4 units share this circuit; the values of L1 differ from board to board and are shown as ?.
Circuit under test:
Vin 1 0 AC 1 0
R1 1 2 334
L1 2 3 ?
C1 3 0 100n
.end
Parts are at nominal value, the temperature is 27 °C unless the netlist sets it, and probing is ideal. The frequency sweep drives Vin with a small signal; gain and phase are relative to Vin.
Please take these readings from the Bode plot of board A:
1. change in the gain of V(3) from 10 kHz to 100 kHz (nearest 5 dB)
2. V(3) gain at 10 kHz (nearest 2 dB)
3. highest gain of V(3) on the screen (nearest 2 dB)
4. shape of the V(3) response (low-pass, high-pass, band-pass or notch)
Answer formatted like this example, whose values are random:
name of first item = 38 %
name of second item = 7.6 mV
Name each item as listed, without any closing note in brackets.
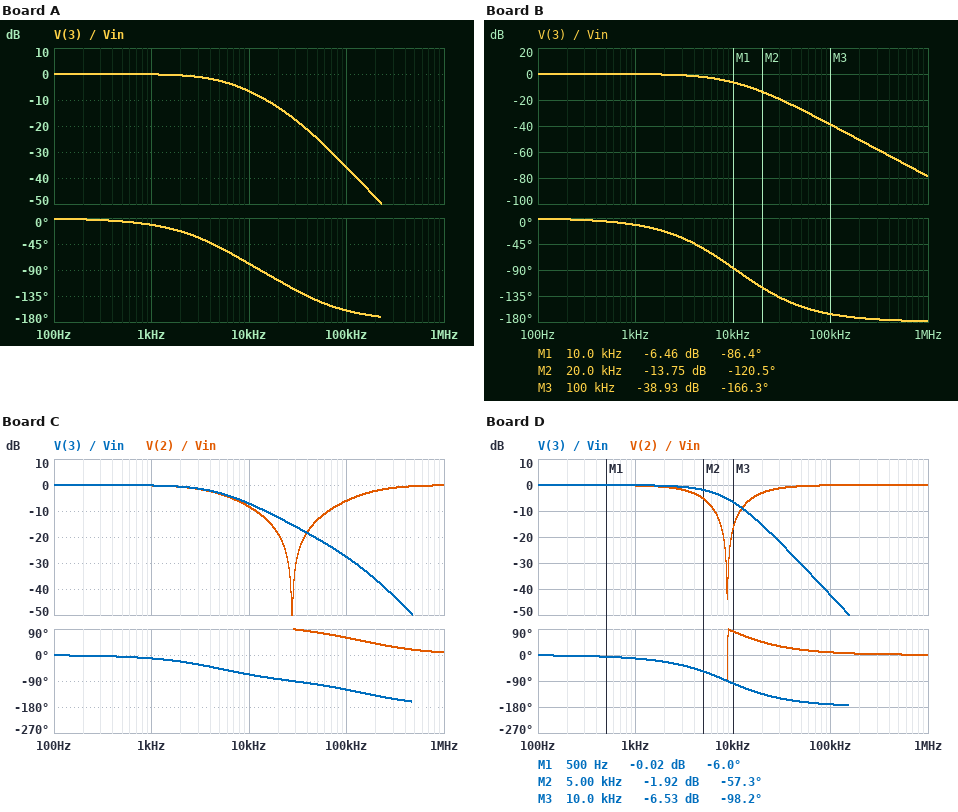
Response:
change in the gain of V(3) from 10 kHz to 100 kHz = -30 dB
V(3) gain at 10 kHz = -6 dB
highest gain of V(3) on the screen = 0 dB
shape of the V(3) response = low-pass
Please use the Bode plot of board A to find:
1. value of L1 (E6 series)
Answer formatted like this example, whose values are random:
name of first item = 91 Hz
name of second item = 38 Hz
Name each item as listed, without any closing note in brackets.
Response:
value of L1 = 1.5 mH
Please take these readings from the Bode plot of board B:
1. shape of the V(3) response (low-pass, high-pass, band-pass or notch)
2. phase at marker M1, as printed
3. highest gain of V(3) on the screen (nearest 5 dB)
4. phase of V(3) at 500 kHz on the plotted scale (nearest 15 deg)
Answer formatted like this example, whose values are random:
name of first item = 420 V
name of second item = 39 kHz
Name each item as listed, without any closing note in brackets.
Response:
shape of the V(3) response = low-pass
phase at marker M1, as printed = -86.4 deg
highest gain of V(3) on the screen = 0 dB
phase of V(3) at 500 kHz on the plotted scale = -180 deg
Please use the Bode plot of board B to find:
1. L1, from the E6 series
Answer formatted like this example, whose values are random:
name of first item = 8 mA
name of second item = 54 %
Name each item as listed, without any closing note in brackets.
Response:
L1, from the E6 series = 2.2 mH
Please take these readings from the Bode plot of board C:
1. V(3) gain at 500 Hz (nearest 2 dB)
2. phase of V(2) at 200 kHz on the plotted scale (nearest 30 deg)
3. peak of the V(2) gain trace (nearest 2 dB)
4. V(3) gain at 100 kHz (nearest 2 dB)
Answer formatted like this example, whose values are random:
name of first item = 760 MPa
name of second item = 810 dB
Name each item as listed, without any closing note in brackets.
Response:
V(3) gain at 500 Hz = 0 dB
phase of V(2) at 200 kHz on the plotted scale = 30 deg
peak of the V(2) gain trace = 0 dB
V(3) gain at 100 kHz = -28 dB
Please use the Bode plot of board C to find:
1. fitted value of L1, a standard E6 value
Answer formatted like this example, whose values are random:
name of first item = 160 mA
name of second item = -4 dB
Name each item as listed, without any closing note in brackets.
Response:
fitted value of L1, a standard E6 value = 330 µH
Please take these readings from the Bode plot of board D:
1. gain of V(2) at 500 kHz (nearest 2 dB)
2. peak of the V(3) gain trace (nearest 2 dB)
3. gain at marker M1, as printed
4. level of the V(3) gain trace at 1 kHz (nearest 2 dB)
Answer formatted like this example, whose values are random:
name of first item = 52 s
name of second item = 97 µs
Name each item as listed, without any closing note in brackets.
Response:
gain of V(2) at 500 kHz = 0 dB
peak of the V(3) gain trace = 0 dB
gain at marker M1, as printed = -0.02 dB
level of the V(3) gain trace at 1 kHz = 0 dB
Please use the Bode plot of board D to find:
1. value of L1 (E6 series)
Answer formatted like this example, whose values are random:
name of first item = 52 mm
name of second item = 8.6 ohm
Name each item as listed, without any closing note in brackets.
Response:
value of L1 = 3.3 mH
